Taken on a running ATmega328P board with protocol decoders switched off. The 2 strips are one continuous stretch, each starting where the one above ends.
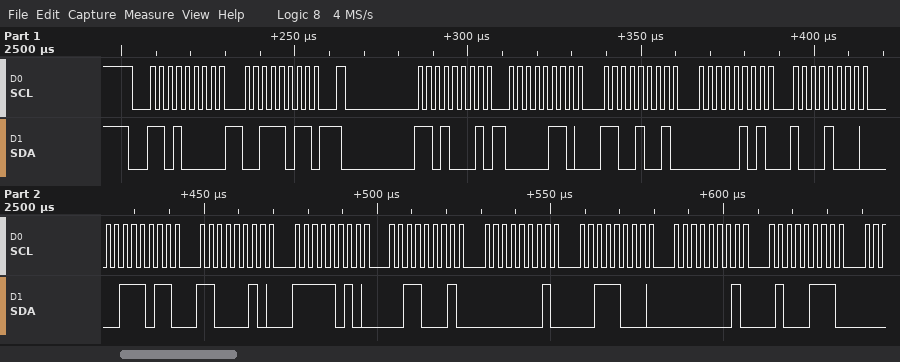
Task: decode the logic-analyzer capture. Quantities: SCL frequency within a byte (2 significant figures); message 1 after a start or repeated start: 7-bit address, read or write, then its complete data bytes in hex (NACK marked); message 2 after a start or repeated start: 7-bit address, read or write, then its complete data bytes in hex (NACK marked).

400 kHz
0x68 write: 3B
0x68 read: 06 C9 05 88 3B C2 FA 31 01 38 01 47
